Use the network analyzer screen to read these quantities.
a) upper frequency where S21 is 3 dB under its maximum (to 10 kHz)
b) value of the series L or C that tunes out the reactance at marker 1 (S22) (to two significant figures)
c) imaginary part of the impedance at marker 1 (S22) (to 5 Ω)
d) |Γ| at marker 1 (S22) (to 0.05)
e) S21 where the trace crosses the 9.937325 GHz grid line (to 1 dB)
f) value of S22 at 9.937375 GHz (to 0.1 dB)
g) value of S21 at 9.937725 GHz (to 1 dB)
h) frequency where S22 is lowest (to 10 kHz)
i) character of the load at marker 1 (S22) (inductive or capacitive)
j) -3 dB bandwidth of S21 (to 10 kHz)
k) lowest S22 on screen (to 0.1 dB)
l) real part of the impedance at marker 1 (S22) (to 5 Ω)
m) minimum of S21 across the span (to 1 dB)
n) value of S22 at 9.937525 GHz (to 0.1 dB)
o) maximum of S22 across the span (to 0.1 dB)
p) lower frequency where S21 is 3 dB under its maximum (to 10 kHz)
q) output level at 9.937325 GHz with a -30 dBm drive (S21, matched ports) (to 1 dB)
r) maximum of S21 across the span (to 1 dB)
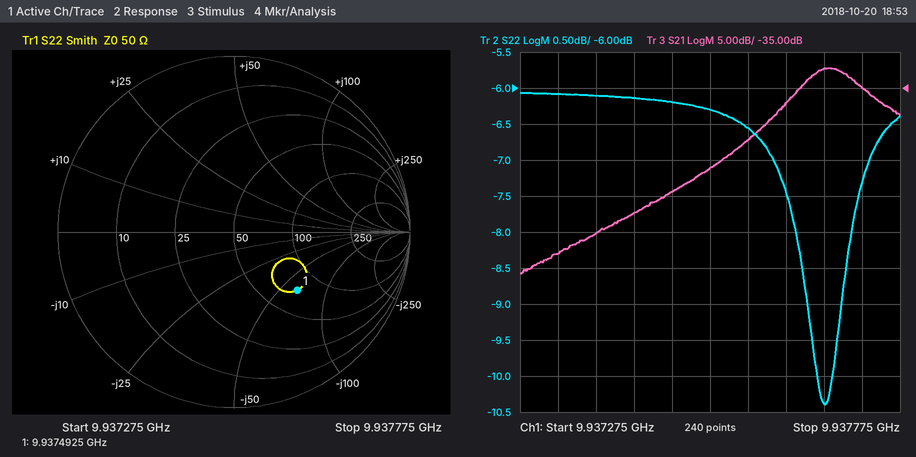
9.93773 GHz
1.0 nH
-65 Ω
0.50
-58 dB
-6.1 dB
-35 dB
9.93768 GHz
capacitive
90 kHz
-10.4 dB
75 Ω
-61 dB
-6.3 dB
-6.1 dB
9.93764 GHz
-88 dBm
-32 dB
